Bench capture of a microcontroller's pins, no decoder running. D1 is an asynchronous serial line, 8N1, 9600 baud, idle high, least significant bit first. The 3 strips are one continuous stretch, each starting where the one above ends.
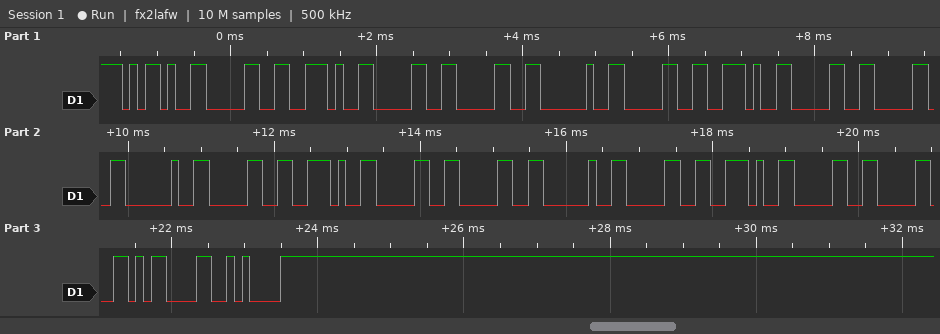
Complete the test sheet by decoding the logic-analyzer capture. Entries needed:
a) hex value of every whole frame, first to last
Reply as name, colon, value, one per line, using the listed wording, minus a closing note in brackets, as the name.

hex value of every whole frame, first to last: 0x2D 0x30 0x2E 0x30 0x30 0x20 0x30 0x2E 0x30 0x30 0x20 0x30 0x2E 0x30 0x30 0x20 0x30 0x2E 0x30 0x30 0x0D 0x0A
